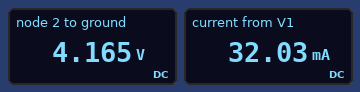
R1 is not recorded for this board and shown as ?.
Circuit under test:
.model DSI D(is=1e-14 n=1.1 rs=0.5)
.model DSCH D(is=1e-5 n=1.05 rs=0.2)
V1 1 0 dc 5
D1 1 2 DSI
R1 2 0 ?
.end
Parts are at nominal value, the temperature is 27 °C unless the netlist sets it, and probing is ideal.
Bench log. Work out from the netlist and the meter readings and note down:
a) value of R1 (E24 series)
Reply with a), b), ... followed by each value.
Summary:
a) 130 Ω
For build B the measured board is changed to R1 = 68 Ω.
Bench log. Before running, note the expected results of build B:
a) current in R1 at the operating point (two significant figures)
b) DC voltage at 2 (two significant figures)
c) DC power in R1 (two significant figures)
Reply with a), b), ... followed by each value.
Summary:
a) 61 mA
b) 4.1 V
c) 250 mW
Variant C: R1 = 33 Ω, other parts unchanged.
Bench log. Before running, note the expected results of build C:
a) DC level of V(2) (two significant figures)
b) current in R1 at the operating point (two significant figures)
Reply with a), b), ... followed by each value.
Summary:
a) 4.1 V
b) 120 mA
